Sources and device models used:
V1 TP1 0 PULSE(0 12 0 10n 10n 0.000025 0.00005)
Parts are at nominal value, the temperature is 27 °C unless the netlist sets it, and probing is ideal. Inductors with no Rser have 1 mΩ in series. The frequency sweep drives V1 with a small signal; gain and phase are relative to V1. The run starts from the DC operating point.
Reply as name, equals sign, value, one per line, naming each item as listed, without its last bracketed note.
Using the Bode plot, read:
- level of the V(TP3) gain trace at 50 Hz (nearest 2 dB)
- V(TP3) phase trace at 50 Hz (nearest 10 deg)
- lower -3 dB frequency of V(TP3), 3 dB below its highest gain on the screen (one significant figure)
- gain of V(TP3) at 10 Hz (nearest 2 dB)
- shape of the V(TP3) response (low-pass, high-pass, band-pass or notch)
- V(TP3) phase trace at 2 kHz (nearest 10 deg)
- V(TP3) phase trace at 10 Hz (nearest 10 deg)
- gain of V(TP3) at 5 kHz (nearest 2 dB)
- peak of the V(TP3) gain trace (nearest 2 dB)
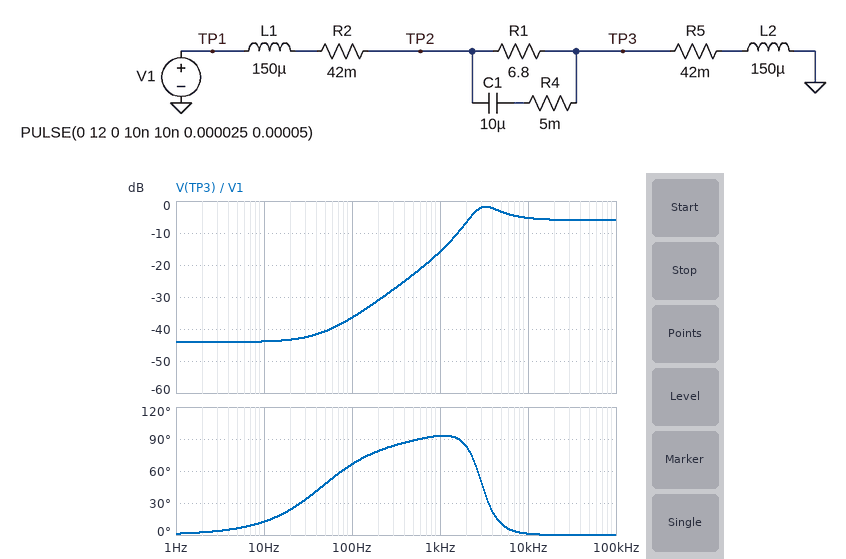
level of the V(TP3) gain trace at 50 Hz = -40 dB
V(TP3) phase trace at 50 Hz = 50 deg
lower -3 dB frequency of V(TP3), 3 dB below its highest gain on the screen = 2 kHz
gain of V(TP3) at 10 Hz = -44 dB
shape of the V(TP3) response = high-pass
V(TP3) phase trace at 2 kHz = 80 deg
V(TP3) phase trace at 10 Hz = 10 deg
gain of V(TP3) at 5 kHz = -4 dB
peak of the V(TP3) gain trace = -2 dB
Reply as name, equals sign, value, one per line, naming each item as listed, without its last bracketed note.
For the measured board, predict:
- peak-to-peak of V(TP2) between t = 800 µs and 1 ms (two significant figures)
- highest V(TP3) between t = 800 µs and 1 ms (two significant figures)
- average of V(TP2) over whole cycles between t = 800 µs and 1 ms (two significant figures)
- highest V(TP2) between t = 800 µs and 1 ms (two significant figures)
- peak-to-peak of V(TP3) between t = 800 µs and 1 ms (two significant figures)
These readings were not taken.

peak-to-peak of V(TP2) between t = 800 µs and 1 ms = 6.0 V
highest V(TP3) between t = 800 µs and 1 ms = 3.1 V
average of V(TP2) over whole cycles between t = 800 µs and 1 ms = 6.0 V
highest V(TP2) between t = 800 µs and 1 ms = 9.0 V
peak-to-peak of V(TP3) between t = 800 µs and 1 ms = 6.2 V
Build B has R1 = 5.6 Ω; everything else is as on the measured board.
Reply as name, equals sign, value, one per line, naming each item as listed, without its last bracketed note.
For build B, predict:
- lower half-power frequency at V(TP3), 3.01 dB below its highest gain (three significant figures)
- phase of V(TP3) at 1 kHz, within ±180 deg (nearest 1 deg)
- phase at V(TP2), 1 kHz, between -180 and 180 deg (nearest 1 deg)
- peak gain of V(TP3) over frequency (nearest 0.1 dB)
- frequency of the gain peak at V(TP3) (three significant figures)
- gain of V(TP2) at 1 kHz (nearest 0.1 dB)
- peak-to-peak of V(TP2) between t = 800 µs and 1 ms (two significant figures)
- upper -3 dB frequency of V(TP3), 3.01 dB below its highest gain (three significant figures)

lower half-power frequency at V(TP3), 3.01 dB below its highest gain = 2.14 kHz
phase of V(TP3) at 1 kHz, within ±180 deg = 86 deg
phase at V(TP2), 1 kHz, between -180 and 180 deg = -11 deg
peak gain of V(TP3) over frequency = -2.7 dB
frequency of the gain peak at V(TP3) = 3.42 kHz
gain of V(TP2) at 1 kHz = 0 dB
peak-to-peak of V(TP2) between t = 800 µs and 1 ms = 6.0 V
upper -3 dB frequency of V(TP3), 3.01 dB below its highest gain = 15.0 kHz
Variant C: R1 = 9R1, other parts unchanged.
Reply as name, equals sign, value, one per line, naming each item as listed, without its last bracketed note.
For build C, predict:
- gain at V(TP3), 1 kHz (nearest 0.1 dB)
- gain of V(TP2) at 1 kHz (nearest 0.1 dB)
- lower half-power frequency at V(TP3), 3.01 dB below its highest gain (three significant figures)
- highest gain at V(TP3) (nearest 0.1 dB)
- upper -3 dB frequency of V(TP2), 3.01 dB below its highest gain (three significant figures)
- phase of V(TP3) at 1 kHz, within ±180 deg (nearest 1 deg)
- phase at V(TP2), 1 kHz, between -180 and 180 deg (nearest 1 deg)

gain at V(TP3), 1 kHz = -17.7 dB
gain of V(TP2) at 1 kHz = 0.3 dB
lower half-power frequency at V(TP3), 3.01 dB below its highest gain = 2.39 kHz
highest gain at V(TP3) = -0.2 dB
upper -3 dB frequency of V(TP2), 3.01 dB below its highest gain = 3.07 kHz
phase of V(TP3) at 1 kHz, within ±180 deg = 104 deg
phase at V(TP2), 1 kHz, between -180 and 180 deg = -7 deg
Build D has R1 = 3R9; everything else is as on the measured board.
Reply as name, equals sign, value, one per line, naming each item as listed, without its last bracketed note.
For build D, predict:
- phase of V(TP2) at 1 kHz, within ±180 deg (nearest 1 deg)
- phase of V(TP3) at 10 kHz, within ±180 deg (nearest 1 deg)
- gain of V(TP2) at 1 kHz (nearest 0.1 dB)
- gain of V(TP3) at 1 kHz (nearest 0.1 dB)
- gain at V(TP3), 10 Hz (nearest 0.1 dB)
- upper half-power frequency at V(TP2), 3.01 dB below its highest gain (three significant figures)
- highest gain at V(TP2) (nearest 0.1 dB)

phase of V(TP2) at 1 kHz, within ±180 deg = -14 deg
phase of V(TP3) at 10 kHz, within ±180 deg = 2 deg
gain of V(TP2) at 1 kHz = -0.4 dB
gain of V(TP3) at 1 kHz = -12.3 dB
gain at V(TP3), 10 Hz = -39.1 dB
upper half-power frequency at V(TP2), 3.01 dB below its highest gain = 2.53 kHz
highest gain at V(TP2) = -0.1 dB
